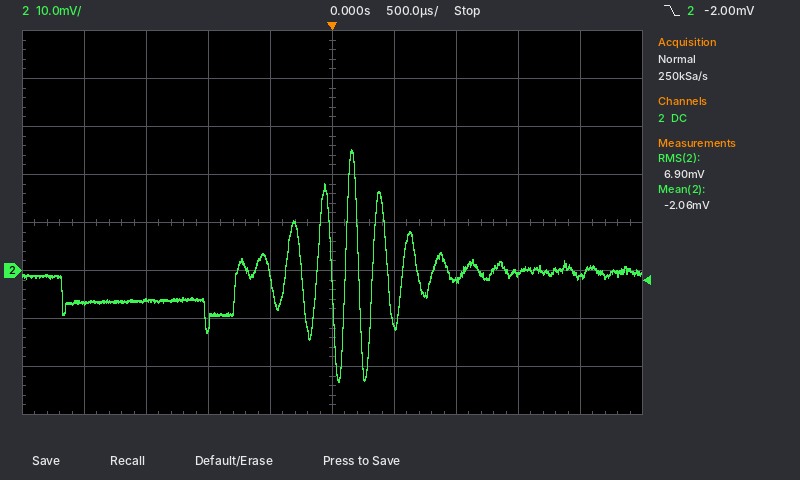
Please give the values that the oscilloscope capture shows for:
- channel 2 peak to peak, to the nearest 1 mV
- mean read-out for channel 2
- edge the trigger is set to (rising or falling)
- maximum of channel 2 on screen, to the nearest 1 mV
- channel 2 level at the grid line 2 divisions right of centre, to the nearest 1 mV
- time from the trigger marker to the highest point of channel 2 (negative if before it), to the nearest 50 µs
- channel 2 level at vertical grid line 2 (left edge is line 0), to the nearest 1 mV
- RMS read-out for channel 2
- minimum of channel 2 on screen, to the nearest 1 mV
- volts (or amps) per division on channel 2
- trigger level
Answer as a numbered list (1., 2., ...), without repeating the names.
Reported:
1. 48 mV
2. -2.06 mV
3. falling
4. 25 mV
5. -2 mV
6. +150 µs
7. -6 mV
8. 6.90 mV
9. -23 mV
10. 10 mV
11. -2.00 mV
